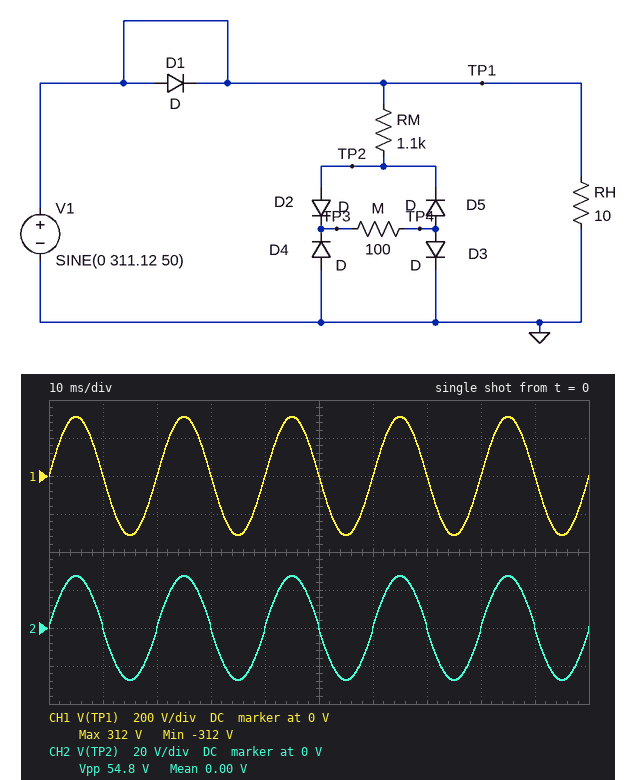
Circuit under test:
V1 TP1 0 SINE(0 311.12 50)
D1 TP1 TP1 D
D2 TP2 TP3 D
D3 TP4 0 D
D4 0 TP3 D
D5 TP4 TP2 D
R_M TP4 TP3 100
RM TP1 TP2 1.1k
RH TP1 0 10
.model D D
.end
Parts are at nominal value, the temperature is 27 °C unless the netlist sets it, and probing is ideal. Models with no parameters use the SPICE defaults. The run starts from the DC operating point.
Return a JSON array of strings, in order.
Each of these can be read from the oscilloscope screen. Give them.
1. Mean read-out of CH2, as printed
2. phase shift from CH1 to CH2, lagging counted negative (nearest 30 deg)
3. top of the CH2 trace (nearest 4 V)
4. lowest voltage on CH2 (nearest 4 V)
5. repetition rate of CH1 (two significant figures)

["0.00 V", "0 deg", "28 V", "-28 V", "50 Hz"]
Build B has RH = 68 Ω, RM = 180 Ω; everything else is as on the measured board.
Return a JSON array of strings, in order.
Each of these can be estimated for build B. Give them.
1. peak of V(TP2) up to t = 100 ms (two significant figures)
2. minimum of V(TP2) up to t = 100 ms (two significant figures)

["110 V", "-110 V"]
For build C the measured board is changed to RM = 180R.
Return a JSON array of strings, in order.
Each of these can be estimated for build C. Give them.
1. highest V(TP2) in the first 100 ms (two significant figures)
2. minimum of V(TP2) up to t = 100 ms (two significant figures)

["110 V", "-110 V"]
